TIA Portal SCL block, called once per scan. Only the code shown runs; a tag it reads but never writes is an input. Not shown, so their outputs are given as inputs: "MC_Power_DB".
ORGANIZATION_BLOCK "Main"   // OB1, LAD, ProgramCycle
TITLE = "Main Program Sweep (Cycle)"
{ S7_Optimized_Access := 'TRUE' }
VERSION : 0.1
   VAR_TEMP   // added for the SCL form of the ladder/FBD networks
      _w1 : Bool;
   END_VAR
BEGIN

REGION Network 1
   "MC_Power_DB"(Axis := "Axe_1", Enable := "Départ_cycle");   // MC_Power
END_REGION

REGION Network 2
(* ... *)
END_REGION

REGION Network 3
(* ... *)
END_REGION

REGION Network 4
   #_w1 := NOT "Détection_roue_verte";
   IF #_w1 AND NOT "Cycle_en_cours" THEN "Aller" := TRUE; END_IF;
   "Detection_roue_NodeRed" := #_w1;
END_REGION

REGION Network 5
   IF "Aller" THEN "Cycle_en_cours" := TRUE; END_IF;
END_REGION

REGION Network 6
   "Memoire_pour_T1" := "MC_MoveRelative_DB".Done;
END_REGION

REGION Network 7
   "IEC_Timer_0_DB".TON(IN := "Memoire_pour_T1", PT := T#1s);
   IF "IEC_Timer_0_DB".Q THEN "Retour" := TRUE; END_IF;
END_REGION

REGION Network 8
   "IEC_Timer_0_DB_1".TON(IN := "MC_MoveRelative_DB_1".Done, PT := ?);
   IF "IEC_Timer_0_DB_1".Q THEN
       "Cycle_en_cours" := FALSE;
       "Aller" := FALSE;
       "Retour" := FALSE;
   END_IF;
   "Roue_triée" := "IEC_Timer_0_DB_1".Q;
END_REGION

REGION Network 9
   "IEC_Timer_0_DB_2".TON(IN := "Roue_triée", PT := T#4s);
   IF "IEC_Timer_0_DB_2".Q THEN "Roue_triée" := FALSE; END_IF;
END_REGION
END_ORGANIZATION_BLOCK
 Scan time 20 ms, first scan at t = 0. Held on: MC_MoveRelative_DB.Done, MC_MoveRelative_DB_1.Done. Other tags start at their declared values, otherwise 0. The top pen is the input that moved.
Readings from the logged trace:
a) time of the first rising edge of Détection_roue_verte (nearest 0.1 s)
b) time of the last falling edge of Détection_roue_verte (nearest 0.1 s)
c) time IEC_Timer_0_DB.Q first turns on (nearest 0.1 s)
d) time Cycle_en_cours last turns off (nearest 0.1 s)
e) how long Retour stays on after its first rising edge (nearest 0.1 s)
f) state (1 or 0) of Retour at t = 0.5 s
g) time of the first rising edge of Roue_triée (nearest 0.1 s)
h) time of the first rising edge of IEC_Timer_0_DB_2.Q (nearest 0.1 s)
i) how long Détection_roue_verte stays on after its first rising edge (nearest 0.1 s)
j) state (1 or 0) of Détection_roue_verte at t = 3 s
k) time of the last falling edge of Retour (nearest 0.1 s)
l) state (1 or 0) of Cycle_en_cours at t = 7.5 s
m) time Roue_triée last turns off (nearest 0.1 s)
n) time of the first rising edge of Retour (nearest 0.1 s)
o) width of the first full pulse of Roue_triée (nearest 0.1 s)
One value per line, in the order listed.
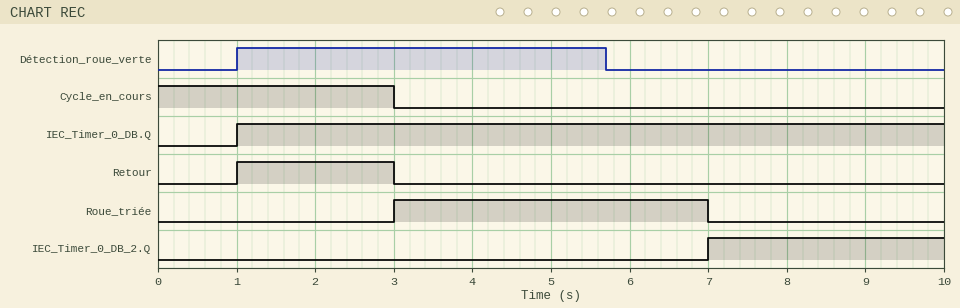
1.0 s
5.7 s
1.0 s
3.0 s
2.0 s
0
3.0 s
7.0 s
4.7 s
1
3.0 s
0
7.0 s
1.0 s
4.0 s
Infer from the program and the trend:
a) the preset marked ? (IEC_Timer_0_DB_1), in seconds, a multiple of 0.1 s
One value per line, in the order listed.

3.0 s
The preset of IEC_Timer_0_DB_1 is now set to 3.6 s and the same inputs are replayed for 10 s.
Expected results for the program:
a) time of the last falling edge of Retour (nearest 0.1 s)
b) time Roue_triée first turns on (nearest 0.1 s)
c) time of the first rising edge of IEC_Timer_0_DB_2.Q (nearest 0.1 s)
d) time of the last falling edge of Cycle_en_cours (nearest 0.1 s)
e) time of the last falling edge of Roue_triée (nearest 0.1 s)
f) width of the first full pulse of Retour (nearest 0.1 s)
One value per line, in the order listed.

3.6 s
3.6 s
7.6 s
3.6 s
7.6 s
2.6 s
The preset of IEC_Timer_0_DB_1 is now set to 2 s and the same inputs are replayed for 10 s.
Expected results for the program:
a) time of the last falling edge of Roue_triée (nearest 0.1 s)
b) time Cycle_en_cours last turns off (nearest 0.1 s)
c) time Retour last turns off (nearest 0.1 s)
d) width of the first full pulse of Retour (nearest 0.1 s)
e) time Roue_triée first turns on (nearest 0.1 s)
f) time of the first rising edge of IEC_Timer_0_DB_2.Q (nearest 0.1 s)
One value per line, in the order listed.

6.0 s
2.0 s
2.0 s
1.0 s
2.0 s
6.0 s
